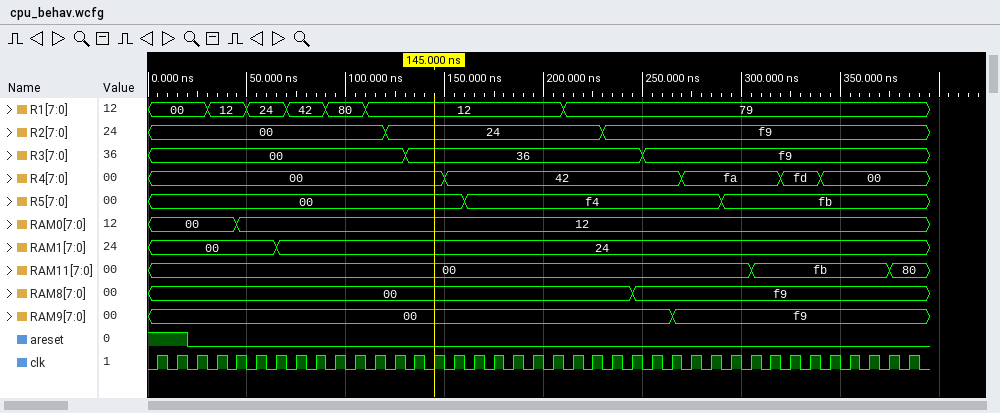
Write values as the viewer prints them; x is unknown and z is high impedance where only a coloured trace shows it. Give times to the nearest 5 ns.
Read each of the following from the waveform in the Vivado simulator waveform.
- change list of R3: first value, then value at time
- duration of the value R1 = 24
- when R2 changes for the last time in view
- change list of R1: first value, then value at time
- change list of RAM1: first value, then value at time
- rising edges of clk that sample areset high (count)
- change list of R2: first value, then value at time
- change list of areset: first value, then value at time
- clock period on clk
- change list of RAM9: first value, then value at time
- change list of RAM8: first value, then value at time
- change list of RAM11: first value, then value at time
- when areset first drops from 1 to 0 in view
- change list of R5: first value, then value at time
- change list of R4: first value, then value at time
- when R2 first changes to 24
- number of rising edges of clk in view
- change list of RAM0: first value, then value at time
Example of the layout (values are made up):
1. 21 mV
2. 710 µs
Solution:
1. 00, 36 at 130 ns, f9 at 250 ns
2. 20 ns
3. 230 ns
4. 00, 12 at 30 ns, 24 at 50 ns, 42 at 70 ns, 80 at 90 ns, 12 at 110 ns, 79 at 210 ns
5. 00, 24 at 65 ns
6. 2
7. 00, 24 at 120 ns, f9 at 230 ns
8. 1, 0 at 20 ns
9. 10 ns
10. 00, f9 at 265 ns
11. 00, f9 at 245 ns
12. 00, fb at 305 ns, 80 at 375 ns
13. 20 ns
14. 00, f4 at 160 ns, fb at 290 ns
15. 00, 42 at 150 ns, fa at 270 ns, fd at 320 ns, 00 at 340 ns
16. 120 ns
17. 39
18. 00, 12 at 45 ns
